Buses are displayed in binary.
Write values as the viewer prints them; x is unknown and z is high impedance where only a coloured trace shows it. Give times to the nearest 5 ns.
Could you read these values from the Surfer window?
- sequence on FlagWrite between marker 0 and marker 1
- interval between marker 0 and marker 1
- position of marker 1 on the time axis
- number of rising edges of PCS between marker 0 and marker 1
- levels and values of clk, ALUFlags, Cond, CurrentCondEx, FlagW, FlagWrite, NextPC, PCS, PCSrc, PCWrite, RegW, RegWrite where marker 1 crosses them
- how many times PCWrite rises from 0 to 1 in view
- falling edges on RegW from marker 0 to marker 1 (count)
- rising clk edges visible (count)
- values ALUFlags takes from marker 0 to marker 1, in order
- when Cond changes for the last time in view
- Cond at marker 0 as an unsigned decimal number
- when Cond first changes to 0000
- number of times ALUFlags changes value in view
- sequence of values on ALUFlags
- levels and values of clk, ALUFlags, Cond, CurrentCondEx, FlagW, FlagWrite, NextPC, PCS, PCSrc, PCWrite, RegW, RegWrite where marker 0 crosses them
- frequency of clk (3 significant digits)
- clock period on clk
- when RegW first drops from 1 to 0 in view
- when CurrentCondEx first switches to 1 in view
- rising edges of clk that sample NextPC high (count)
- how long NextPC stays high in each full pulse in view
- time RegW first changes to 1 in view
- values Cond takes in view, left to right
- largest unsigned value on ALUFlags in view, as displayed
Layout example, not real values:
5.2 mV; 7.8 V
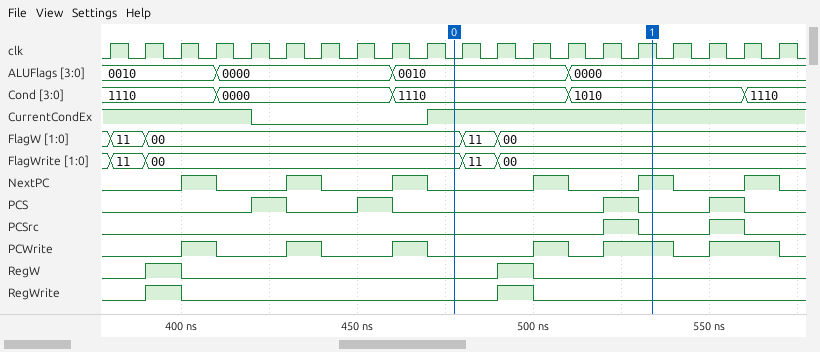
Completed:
00, 11, 00; 55 ns; 535 ns; 1; clk=1, ALUFlags=0000, Cond=1010, CurrentCondEx=1, FlagW=00, FlagWrite=00, NextPC=1, PCS=0, PCSrc=0, PCWrite=1, RegW=0, RegWrite=0; 6; 1; 20; 0010, 0000; 560 ns; 14; 410 ns; 3; 0010, 0000, 0010, 0000; clk=0, ALUFlags=0010, Cond=1110, CurrentCondEx=1, FlagW=00, FlagWrite=00, NextPC=0, PCS=0, PCSrc=0, PCWrite=0, RegW=0, RegWrite=0; 100 MHz; 10 ns; 400 ns; 470 ns; 6; 10 ns, 10 ns, 10 ns, 10 ns, 10 ns, 10 ns; 390 ns; 1110, 0000, 1110, 1010, 1110; 0010
